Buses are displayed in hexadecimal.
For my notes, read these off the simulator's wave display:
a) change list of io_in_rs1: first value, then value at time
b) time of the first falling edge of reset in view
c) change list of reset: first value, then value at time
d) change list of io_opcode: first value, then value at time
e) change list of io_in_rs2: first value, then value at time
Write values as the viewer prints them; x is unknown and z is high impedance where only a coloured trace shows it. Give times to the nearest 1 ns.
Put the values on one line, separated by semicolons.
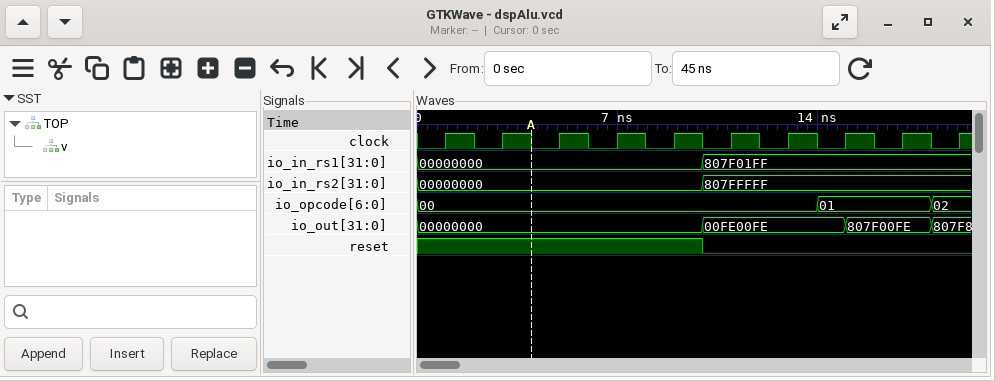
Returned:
00000000, 807F01FF at 10 ns; 10 ns; 1, 0 at 10 ns; 00, 01 at 14 ns, 02 at 18 ns; 00000000, 807FFFFF at 10 ns
